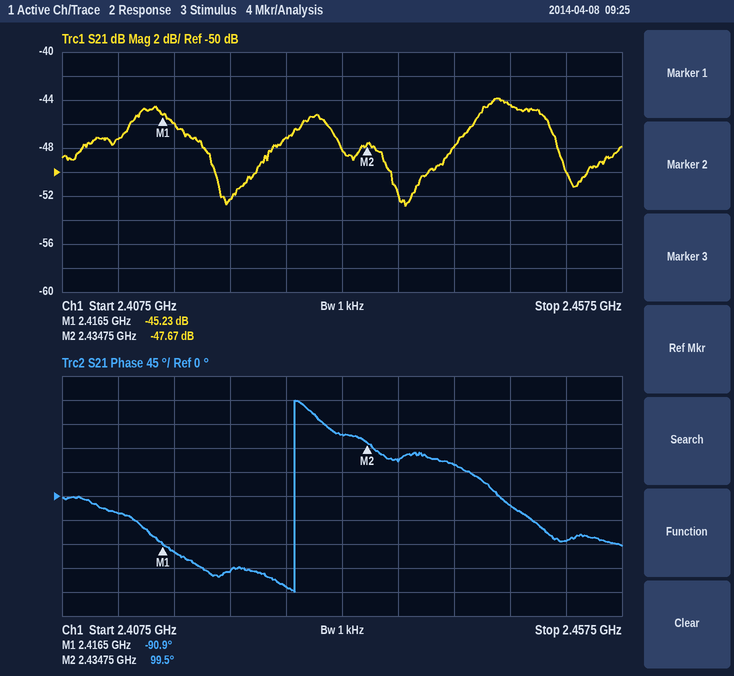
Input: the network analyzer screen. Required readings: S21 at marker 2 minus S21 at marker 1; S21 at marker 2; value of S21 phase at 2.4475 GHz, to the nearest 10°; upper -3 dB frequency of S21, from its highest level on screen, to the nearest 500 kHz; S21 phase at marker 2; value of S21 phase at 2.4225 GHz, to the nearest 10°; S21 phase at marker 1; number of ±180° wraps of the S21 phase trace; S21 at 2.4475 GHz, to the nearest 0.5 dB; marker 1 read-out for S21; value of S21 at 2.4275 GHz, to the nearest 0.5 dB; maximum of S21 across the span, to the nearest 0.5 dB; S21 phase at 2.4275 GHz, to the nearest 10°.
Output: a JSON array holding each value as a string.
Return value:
["-2.44 dB", "-47.67 dB", "-20°", "2.4515 GHz", "99.5°", "-140°", "-90.9°", "1", "-44.5 dB", "-45.23 dB", "-47.0 dB", "-44.0 dB", "-170°"]
